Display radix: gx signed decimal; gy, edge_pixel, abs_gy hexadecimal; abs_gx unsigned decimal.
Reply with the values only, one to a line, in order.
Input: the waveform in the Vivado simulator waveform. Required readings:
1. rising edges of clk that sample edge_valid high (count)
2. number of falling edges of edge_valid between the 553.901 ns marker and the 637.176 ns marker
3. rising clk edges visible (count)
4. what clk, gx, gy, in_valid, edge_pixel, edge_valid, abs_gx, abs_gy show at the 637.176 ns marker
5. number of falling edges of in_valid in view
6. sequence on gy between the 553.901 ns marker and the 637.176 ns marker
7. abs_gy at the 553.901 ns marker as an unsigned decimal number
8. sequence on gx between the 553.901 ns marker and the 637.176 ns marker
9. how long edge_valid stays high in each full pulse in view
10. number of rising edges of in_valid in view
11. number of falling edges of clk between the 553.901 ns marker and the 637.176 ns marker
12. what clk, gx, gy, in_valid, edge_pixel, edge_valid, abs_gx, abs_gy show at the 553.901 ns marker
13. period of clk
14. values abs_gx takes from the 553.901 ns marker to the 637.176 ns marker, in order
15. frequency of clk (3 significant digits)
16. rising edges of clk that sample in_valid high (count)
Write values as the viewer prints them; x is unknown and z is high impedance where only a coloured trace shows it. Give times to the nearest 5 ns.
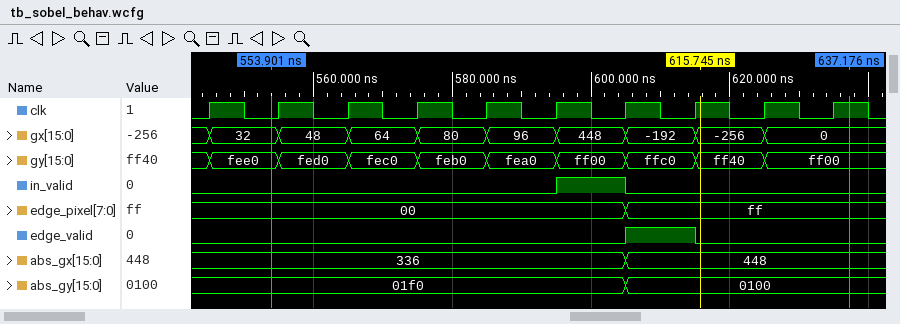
1
1
10
clk=1, gx=0, gy=ff00, in_valid=0, edge_pixel=ff, edge_valid=0, abs_gx=448, abs_gy=0100
1
fee0, fed0, fec0, feb0, fea0, ff00, ffc0, ff40, ff00
496
32, 48, 64, 80, 96, 448, -192, -256, 0
10 ns
1
8
clk=0, gx=32, gy=fee0, in_valid=0, edge_pixel=00, edge_valid=0, abs_gx=336, abs_gy=01f0
10 ns
336, 448
100 MHz
1
